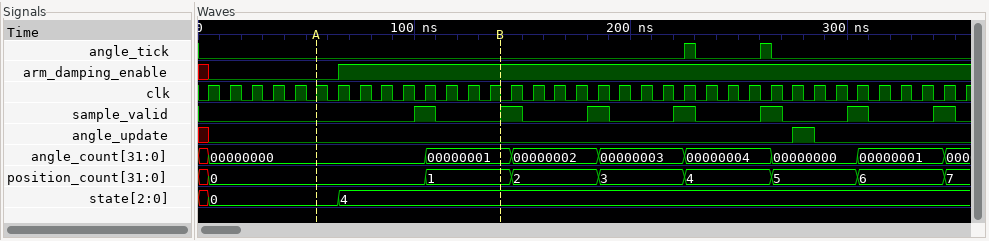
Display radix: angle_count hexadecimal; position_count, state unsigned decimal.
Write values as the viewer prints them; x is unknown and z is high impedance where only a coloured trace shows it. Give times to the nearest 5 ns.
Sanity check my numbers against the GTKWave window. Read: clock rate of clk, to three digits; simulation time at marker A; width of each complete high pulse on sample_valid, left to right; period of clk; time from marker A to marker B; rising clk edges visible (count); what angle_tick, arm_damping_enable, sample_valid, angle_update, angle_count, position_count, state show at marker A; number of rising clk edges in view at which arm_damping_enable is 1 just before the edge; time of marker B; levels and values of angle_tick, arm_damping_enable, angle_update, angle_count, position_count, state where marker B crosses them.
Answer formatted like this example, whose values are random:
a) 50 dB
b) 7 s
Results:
a) 100 MHz
b) 55 ns
c) 10 ns, 10 ns, 10 ns, 10 ns, 10 ns, 10 ns, 10 ns
d) 10 ns
e) 85 ns
f) 36
g) angle_tick=0, arm_damping_enable=0, sample_valid=0, angle_update=0, angle_count=00000000, position_count=0, state=0
h) 29
i) 140 ns
j) angle_tick=0, arm_damping_enable=1, angle_update=0, angle_count=00000001, position_count=1, state=4
